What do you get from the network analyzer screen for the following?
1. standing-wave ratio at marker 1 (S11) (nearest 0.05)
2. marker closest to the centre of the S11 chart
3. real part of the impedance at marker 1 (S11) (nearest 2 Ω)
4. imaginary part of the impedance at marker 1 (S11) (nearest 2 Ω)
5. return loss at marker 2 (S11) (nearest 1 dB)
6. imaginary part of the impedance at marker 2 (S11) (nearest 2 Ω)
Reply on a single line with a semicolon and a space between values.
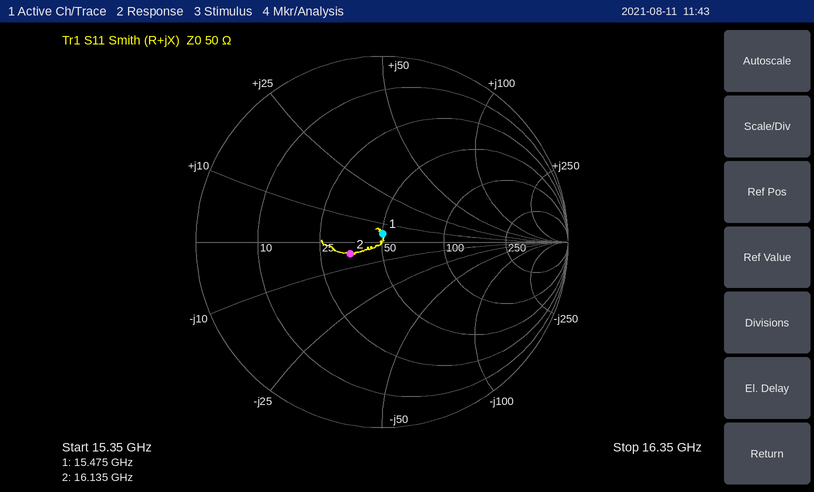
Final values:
1.10; marker 1; 50 Ω; +4 Ω; 15 dB; -4 Ω
